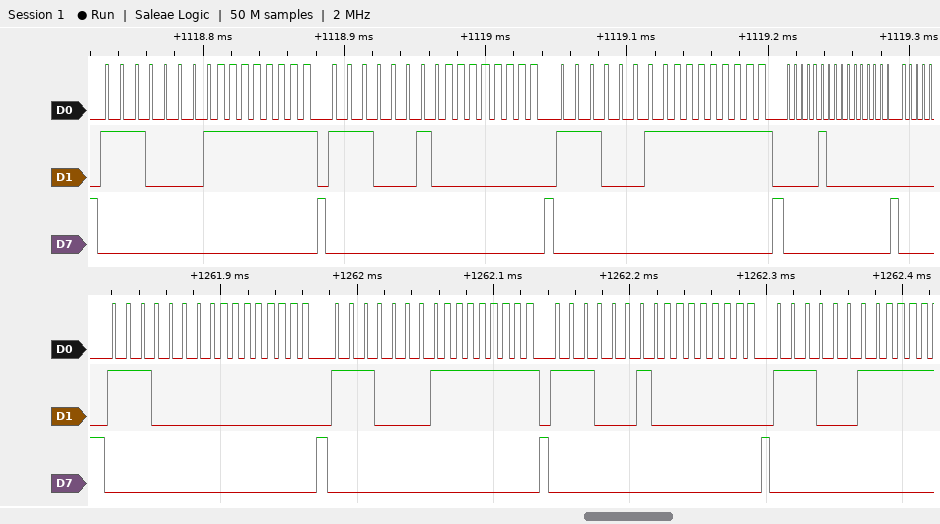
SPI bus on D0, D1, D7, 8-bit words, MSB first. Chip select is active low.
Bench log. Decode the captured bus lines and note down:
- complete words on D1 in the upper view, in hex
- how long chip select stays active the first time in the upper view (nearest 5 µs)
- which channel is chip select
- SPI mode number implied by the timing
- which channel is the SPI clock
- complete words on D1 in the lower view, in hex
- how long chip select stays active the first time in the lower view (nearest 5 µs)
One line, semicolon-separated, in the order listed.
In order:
E1, FF, E2, 00, E3, FF, 04, 00; 155 µs; D7; 1; D0; E0, 00, E1, FF, E2, 00, E3; 155 µs
